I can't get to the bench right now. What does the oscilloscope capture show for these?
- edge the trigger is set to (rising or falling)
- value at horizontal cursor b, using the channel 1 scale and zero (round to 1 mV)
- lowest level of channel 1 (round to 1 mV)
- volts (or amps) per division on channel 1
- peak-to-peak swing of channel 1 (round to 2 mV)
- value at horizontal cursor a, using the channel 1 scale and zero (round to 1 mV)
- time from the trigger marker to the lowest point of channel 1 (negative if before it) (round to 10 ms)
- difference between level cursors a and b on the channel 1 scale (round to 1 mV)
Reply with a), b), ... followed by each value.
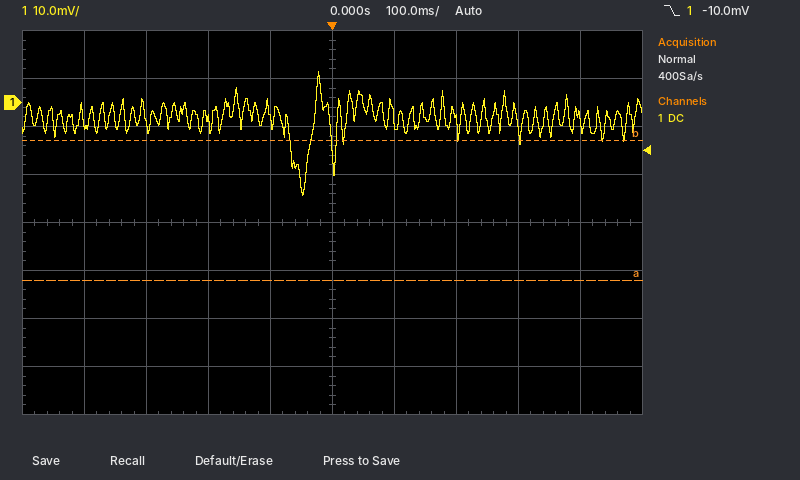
a) falling
b) -8 mV
c) -19 mV
d) 10 mV
e) 26 mV
f) -37 mV
g) -50 ms
h) 29 mV
